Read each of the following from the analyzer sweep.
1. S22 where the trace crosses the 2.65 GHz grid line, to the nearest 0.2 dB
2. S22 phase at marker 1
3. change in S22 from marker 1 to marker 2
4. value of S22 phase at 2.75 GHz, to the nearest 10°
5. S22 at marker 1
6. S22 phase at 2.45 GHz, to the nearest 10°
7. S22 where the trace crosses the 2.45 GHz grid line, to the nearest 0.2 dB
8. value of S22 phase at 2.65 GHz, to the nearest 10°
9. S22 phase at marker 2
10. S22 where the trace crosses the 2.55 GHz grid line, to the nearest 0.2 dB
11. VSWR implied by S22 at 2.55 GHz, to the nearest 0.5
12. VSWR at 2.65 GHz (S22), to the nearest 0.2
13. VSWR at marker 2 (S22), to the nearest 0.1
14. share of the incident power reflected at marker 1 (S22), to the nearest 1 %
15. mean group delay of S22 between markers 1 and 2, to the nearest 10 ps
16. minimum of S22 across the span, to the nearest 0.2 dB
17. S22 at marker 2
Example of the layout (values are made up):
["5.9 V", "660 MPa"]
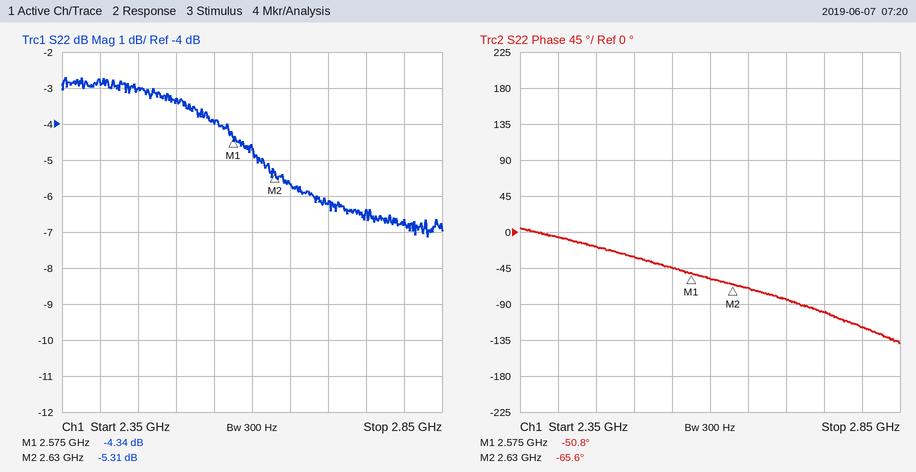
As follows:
["-5.6 dB", "-50.8°", "-0.97 dB", "-100°", "-4.34 dB", "-20°", "-3.0 dB", "-70°", "-65.6°", "-4.0 dB", "4.5", "3.2", "3.4", "37 %", "750 ps", "-7.2 dB", "-5.31 dB"]
